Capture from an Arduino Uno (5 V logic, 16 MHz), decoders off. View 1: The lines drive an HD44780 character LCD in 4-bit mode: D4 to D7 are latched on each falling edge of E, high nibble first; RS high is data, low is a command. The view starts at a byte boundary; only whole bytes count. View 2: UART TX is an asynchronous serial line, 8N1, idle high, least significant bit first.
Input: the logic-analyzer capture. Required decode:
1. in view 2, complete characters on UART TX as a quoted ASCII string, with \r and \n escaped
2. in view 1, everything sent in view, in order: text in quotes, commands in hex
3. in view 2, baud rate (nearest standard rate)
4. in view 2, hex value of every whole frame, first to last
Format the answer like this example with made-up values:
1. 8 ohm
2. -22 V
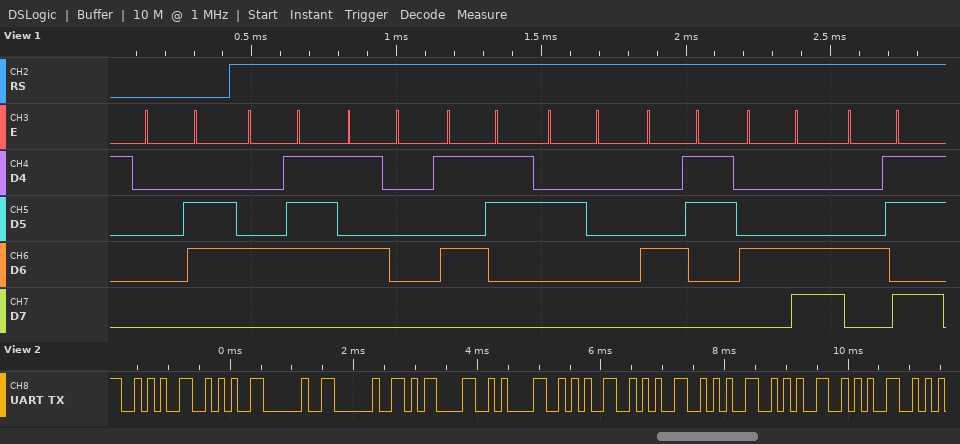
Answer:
1. "**  \r\n*****"
2. 0x06 "GPS CLK"
3. 9600 baud
4. 2A 2A 20 20 0D 0A 2A 2A 2A 2A 2A
